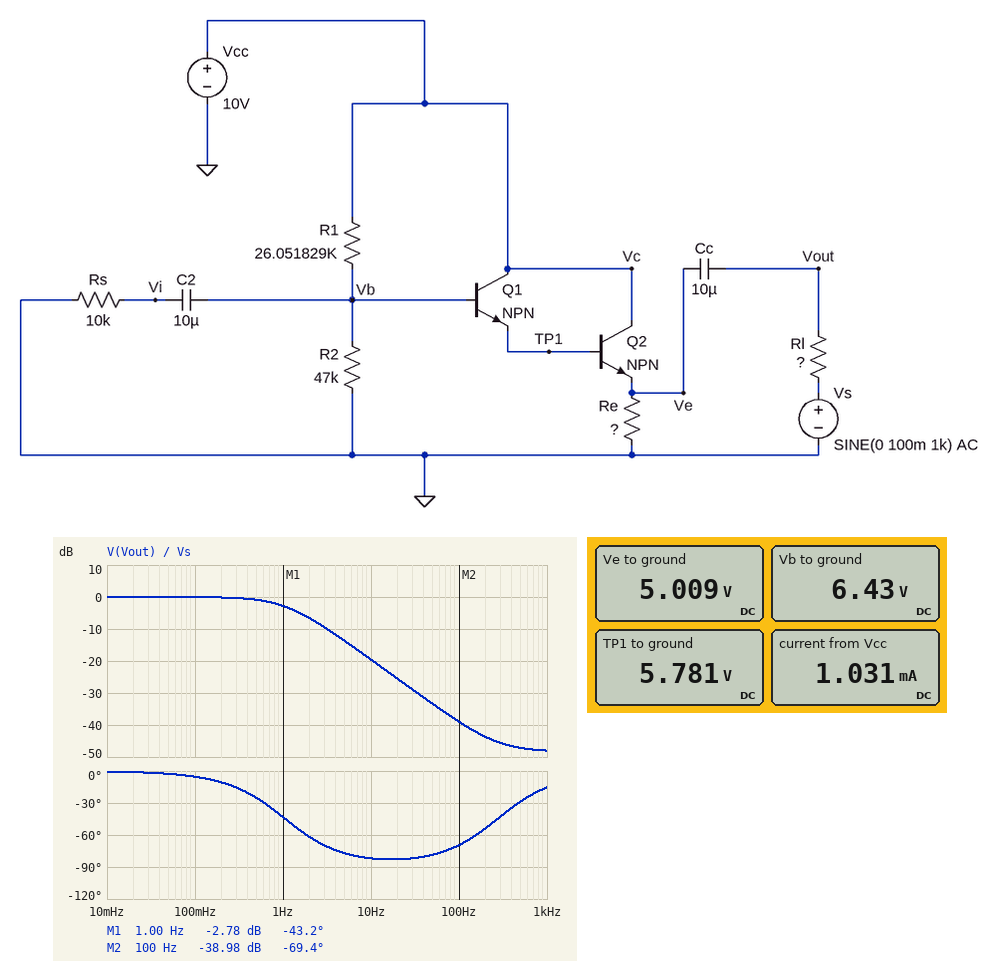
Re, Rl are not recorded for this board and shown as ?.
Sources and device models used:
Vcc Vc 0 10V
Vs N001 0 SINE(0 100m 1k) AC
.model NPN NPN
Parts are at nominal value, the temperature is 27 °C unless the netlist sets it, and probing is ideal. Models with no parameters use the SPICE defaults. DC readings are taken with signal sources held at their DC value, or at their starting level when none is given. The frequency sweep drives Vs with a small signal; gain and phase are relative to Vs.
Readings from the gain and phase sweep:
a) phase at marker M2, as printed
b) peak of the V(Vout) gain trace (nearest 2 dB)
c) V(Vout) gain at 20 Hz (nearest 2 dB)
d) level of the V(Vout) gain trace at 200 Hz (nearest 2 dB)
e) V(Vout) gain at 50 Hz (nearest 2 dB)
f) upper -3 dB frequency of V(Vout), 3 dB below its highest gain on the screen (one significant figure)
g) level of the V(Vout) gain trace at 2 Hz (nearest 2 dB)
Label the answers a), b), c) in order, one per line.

a) -69.4 deg
b) 0 dB
c) -26 dB
d) -44 dB
e) -34 dB
f) 1 Hz
g) -6 dB
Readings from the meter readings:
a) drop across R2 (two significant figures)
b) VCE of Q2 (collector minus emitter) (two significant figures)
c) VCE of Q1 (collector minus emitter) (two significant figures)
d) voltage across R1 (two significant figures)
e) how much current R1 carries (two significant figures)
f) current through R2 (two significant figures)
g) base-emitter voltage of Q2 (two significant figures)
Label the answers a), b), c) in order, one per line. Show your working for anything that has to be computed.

a) 6.43 V = 6.4 V
b) 10 V - 5.009 V = 5.0 V
c) 10 V - 5.781 V = 4.2 V
d) 10 V - 6.43 V = 3.6 V
e) (10 V - 6.43 V) / 26.05 kΩ = 140 µA
f) (6.43 V) / 47 kΩ = 140 µA
g) 5.781 V - 5.009 V = 770 mV
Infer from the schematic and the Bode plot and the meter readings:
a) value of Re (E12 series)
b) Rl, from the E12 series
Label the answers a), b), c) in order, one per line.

a) 5.6 kΩ
b) 15 kΩ
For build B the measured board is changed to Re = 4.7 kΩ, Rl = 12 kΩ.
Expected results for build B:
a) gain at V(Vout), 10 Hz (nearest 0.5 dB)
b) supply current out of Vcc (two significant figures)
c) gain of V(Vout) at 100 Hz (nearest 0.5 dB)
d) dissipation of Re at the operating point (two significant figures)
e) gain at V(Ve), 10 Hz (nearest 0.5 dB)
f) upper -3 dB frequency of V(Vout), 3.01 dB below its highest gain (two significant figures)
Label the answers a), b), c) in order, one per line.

a) -17.5 dB
b) 1.2 mA
c) -37.0 dB
d) 5.3 mW
e) -48.0 dB
f) 1.3 Hz
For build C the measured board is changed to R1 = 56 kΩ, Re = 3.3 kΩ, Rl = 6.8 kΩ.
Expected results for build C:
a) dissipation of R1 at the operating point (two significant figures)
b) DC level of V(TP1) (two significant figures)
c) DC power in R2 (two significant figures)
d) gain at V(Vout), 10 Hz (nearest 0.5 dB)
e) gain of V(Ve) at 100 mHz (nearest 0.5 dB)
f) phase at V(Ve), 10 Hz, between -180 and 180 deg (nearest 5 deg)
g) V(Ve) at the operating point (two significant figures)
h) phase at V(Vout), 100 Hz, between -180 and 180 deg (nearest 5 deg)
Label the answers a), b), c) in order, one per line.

a) 530 µW
b) 3.9 V
c) 440 µW
d) -13.0 dB
e) -69.0 dB
f) 15 deg
g) 3.1 V
h) -70 deg
